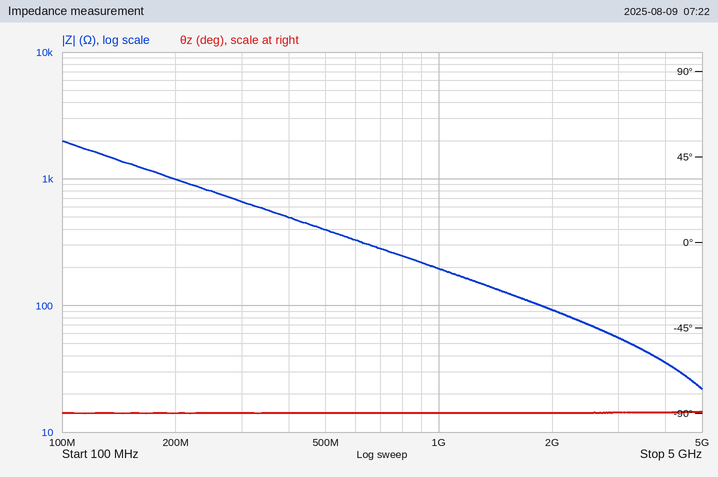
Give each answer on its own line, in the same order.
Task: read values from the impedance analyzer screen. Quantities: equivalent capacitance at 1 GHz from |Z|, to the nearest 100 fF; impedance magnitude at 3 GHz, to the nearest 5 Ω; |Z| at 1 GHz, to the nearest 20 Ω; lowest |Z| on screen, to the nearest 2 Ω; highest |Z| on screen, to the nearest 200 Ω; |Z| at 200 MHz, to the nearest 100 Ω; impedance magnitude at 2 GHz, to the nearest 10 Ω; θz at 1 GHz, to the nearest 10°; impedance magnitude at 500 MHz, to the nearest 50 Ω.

800 fF
55 Ω
200 Ω
22 Ω
2.0 kΩ
1.0 kΩ
90 Ω
-90°
400 Ω
